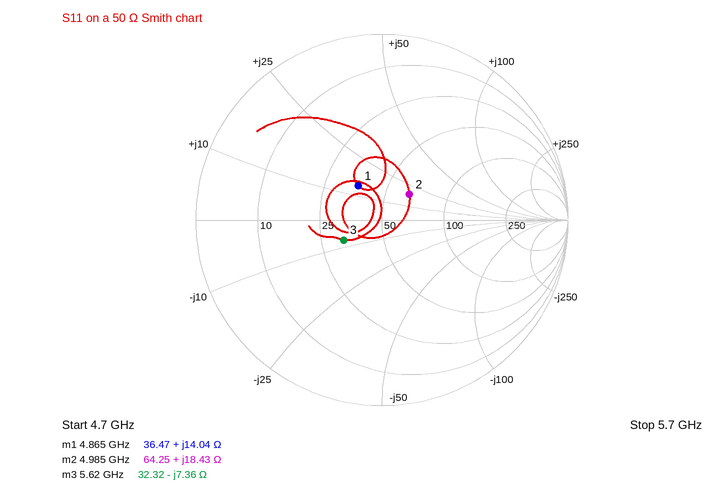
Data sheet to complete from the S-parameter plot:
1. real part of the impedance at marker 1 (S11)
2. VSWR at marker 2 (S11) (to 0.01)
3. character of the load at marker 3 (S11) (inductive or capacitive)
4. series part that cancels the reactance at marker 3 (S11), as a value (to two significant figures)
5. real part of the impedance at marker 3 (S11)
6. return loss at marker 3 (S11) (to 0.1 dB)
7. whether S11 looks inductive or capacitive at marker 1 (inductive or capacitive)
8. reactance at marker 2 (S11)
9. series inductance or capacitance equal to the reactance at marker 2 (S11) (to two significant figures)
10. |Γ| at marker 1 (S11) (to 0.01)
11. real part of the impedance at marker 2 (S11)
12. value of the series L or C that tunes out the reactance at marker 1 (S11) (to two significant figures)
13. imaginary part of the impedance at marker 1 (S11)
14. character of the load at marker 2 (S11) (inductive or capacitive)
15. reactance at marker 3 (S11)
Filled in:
36.47 Ω
1.50
capacitive
210 pH
32.32 Ω
12.7 dB
inductive
+18.43 Ω
590 pH
0.22
64.25 Ω
2.3 pF
+14.04 Ω
inductive
-7.36 Ω
